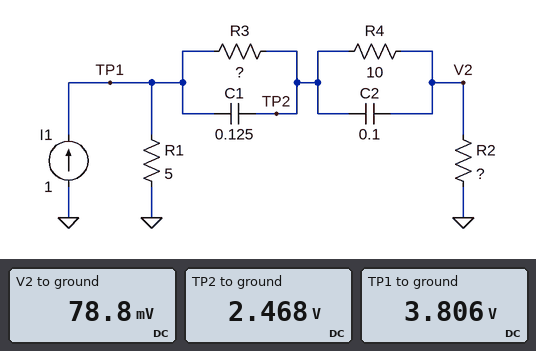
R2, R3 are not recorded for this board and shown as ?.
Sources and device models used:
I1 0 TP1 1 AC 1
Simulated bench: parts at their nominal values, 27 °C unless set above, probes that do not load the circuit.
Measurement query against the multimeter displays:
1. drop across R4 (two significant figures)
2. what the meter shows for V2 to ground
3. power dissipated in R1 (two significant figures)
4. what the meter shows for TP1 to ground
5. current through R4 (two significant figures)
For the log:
2.4 V
78.8 mV
2.9 W
3.806 V
240 mA
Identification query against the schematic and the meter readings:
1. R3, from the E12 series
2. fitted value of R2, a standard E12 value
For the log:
5.6 Ω
0.33 Ω
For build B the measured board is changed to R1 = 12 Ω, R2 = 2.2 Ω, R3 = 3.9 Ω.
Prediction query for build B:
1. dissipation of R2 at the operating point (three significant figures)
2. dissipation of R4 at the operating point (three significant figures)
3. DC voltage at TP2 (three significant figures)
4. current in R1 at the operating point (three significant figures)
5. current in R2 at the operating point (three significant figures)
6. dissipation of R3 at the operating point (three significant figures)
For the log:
401 mW
1.82 W
5.21 V
573 mA
427 mA
711 mW
